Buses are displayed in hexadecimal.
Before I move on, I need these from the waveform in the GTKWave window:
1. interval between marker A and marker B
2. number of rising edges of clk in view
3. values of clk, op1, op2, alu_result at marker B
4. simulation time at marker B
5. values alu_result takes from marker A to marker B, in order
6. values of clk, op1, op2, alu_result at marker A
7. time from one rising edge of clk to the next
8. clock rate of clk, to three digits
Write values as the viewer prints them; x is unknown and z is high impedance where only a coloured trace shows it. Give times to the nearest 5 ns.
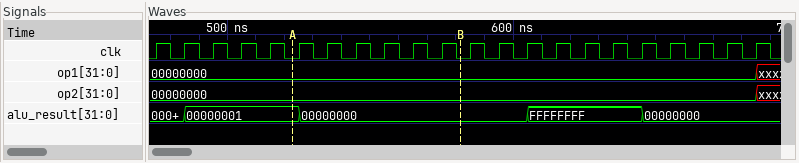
60 ns
22
clk=0, op1=00000000, op2=00000000, alu_result=00000000
580 ns
00000001, 00000000
clk=0, op1=00000000, op2=00000000, alu_result=00000001
10 ns
100 MHz
